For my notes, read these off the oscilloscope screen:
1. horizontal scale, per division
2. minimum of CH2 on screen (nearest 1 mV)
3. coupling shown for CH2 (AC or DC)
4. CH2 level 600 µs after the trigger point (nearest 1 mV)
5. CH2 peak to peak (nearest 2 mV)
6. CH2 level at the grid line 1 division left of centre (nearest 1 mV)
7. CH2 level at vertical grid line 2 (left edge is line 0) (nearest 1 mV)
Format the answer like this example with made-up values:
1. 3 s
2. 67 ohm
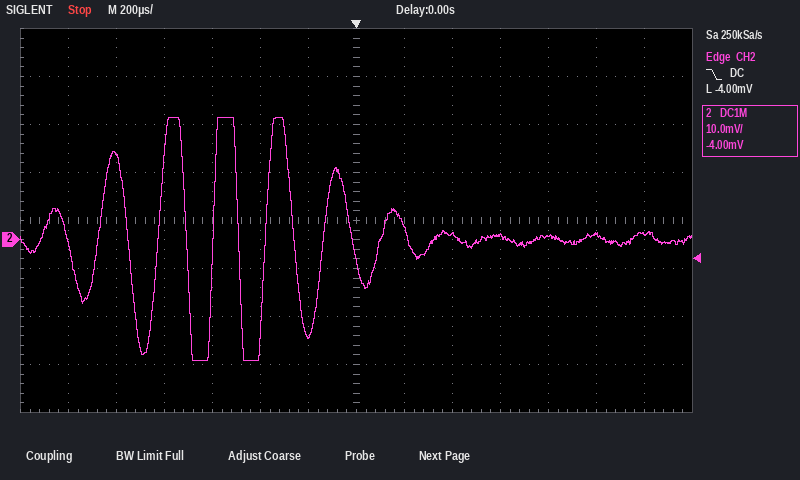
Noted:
1. 200 µs
2. -25 mV
3. DC
4. 1 mV
5. 50 mV
6. -20 mV
7. 18 mV
